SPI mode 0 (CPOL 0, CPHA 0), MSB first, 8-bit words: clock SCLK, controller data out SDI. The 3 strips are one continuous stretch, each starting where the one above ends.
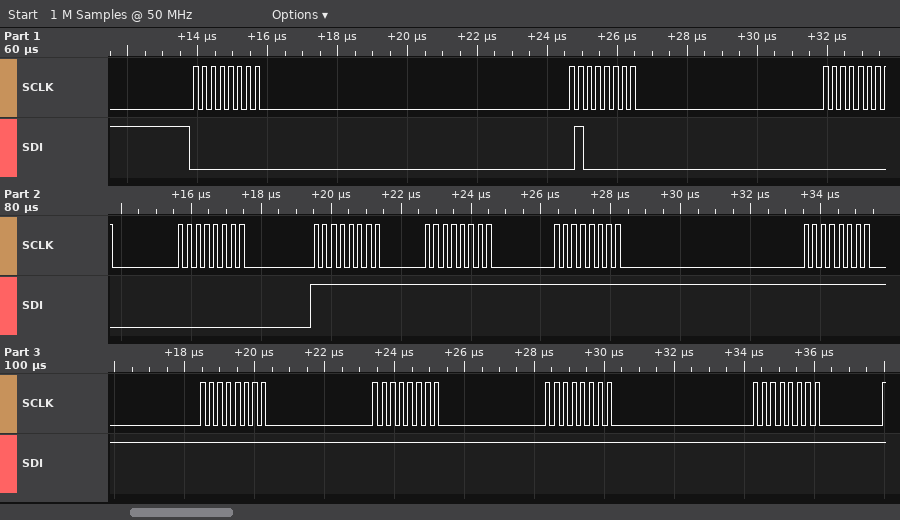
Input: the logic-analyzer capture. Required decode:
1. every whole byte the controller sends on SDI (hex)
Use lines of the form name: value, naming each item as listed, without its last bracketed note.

every whole byte the controller sends on SDI: 00 40 00 00 FF FF FF FF FF FF FF FF
